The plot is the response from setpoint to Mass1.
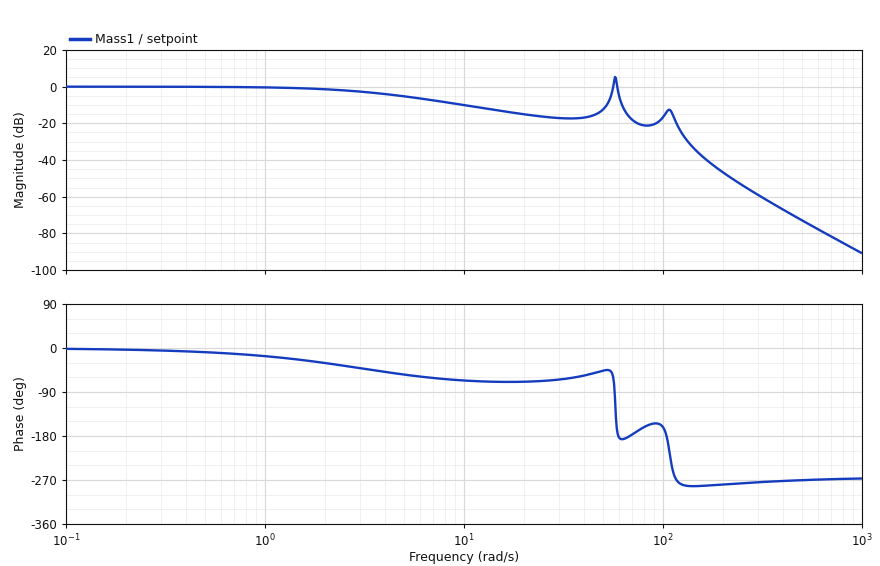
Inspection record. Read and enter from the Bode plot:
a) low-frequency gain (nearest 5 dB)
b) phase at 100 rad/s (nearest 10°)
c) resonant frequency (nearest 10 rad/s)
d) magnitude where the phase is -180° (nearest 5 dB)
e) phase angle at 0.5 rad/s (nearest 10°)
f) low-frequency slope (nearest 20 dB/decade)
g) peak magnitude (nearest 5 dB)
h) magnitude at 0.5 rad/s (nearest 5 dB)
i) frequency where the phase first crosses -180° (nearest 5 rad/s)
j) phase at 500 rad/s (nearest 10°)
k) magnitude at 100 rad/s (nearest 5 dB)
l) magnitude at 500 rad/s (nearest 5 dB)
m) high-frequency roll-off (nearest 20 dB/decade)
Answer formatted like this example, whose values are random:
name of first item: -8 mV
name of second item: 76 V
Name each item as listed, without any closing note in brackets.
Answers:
low-frequency gain: 0 dB
phase at 100 rad/s: -160°
resonant frequency: 60 rad/s
magnitude where the phase is -180°: -5 dB
phase angle at 0.5 rad/s: -10°
low-frequency slope: 0 dB/decade
peak magnitude: 5 dB
magnitude at 0.5 rad/s: 0 dB
frequency where the phase first crosses -180°: 60 rad/s
phase at 500 rad/s: -270°
magnitude at 100 rad/s: -15 dB
magnitude at 500 rad/s: -75 dB
high-frequency roll-off: -60 dB/decade
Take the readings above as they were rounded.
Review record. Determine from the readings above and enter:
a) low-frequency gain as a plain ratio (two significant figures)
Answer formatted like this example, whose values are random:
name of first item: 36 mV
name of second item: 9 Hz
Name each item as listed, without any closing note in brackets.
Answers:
low-frequency gain as a plain ratio: 1.0
